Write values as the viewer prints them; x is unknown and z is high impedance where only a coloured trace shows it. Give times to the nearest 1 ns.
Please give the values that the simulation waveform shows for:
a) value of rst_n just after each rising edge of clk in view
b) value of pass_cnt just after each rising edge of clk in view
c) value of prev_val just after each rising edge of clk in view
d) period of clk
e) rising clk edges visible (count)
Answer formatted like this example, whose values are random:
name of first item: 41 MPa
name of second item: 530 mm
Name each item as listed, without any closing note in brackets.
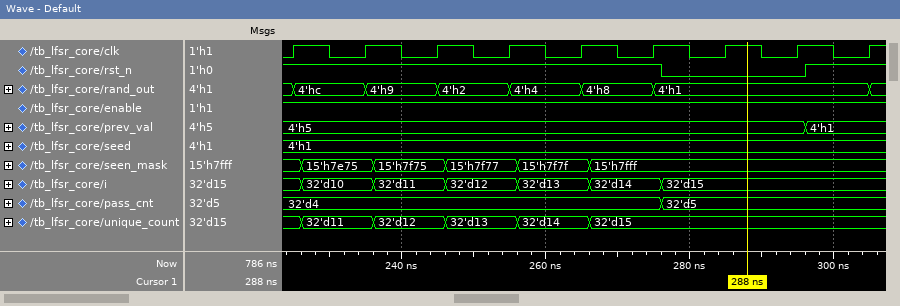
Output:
value of rst_n just after each rising edge of clk in view: 1 1 1 1 1 1 0 0 1
value of pass_cnt just after each rising edge of clk in view: 32'd4, 32'd4, 32'd4, 32'd4, 32'd4, 32'd4, 32'd5, 32'd5, 32'd5
value of prev_val just after each rising edge of clk in view: 4'h5, 4'h5, 4'h5, 4'h5, 4'h5, 4'h5, 4'h5, 4'h5, 4'h1
period of clk: 10 ns
rising clk edges visible: 9
